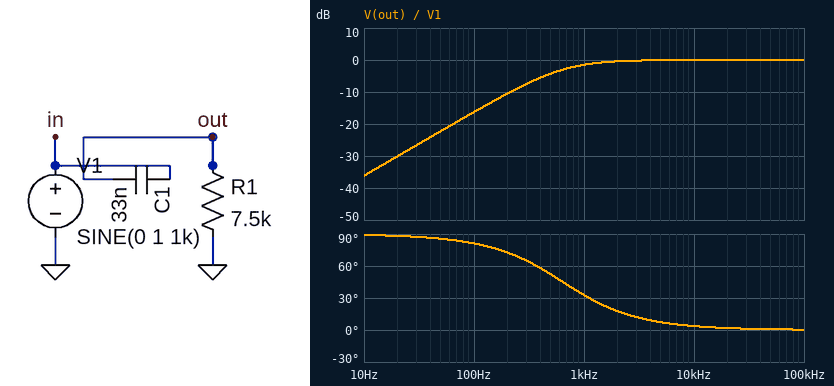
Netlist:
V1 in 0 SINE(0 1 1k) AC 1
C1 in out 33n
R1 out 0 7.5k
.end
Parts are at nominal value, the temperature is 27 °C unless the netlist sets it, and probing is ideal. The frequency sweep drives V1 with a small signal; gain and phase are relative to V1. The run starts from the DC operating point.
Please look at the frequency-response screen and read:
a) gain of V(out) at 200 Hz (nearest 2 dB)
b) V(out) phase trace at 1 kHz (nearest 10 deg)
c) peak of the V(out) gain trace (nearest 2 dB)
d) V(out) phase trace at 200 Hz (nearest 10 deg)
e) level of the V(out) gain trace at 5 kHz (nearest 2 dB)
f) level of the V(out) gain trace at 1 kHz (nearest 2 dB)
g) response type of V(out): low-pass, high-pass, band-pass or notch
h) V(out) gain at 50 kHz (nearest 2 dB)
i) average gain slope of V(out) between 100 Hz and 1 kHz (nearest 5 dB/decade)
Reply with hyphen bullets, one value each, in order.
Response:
- -10 dB
- 30 deg
- 0 dB
- 70 deg
- 0 dB
- -2 dB
- high-pass
- 0 dB
- 15 dB/decade
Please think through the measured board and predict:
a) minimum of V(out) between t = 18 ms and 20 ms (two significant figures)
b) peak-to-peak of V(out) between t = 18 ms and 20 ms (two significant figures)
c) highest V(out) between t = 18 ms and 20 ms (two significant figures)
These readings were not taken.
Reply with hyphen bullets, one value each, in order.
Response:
- -840 mV
- 1.7 V
- 840 mV
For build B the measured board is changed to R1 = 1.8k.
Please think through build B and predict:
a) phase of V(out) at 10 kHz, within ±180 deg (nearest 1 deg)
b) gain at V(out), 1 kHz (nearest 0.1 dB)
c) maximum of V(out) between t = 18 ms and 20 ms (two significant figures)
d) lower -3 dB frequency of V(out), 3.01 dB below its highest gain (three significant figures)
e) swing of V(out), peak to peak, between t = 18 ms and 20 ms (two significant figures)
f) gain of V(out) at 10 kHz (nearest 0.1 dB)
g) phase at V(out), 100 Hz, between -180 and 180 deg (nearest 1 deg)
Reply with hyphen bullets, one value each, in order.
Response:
- 15 deg
- -9.1 dB
- 350 mV
- 2.68 kHz
- 700 mV
- -0.3 dB
- 88 deg
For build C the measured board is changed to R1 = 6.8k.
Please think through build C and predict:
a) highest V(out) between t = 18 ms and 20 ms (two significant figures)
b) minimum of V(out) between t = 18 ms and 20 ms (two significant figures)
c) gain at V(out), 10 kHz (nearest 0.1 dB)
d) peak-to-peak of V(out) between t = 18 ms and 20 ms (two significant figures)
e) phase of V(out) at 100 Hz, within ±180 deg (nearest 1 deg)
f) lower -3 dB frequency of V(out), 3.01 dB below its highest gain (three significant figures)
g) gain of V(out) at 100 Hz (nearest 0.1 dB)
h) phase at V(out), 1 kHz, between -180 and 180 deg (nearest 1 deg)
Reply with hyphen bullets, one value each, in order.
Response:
- 820 mV
- -820 mV
- 0 dB
- 1.6 V
- 82 deg
- 709 Hz
- -17.1 dB
- 35 deg
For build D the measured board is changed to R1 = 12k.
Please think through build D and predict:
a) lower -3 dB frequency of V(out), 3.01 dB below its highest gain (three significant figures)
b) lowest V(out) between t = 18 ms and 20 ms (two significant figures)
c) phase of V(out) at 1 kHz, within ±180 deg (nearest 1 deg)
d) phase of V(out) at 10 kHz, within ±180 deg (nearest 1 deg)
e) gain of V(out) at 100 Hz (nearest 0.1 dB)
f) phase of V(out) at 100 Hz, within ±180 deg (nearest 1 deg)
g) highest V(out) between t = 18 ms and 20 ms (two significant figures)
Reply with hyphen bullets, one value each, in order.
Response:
- 402 Hz
- -930 mV
- 22 deg
- 2 deg
- -12.3 dB
- 76 deg
- 930 mV
